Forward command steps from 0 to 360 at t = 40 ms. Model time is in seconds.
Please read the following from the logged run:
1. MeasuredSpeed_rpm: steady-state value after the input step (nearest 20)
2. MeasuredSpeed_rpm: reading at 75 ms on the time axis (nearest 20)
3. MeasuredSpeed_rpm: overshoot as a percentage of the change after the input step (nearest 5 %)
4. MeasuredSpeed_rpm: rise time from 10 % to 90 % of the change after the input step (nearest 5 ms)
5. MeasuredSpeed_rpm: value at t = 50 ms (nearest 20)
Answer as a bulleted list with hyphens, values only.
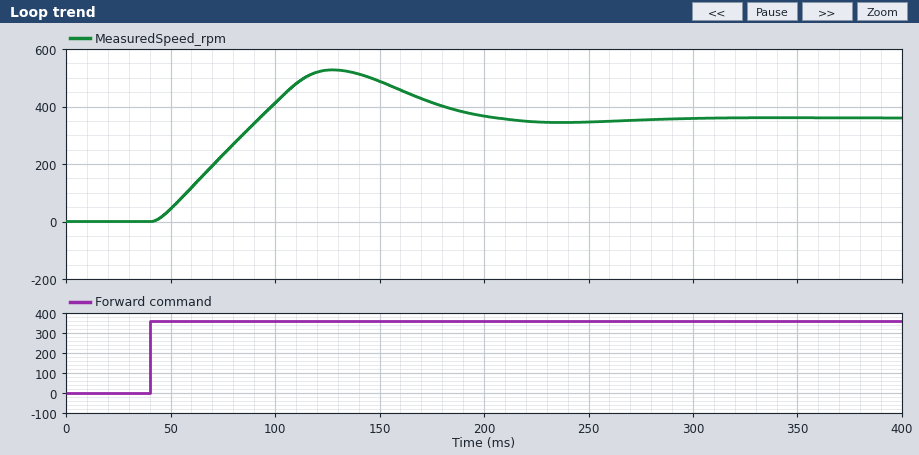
- 360
- 240
- 45 %
- 40 ms
- 40
